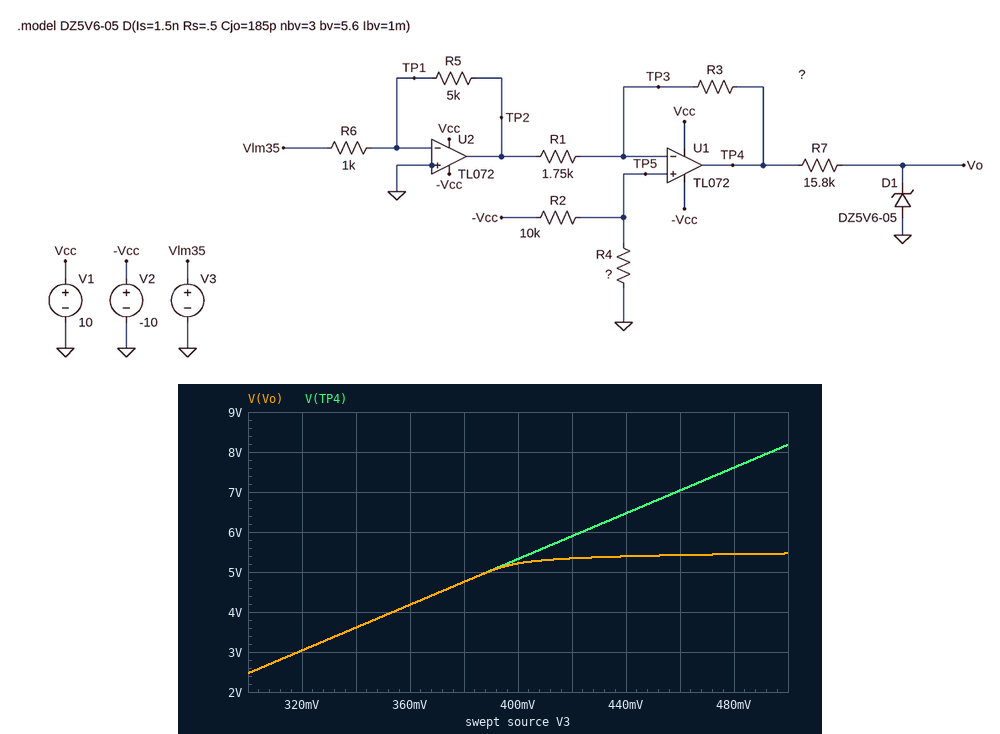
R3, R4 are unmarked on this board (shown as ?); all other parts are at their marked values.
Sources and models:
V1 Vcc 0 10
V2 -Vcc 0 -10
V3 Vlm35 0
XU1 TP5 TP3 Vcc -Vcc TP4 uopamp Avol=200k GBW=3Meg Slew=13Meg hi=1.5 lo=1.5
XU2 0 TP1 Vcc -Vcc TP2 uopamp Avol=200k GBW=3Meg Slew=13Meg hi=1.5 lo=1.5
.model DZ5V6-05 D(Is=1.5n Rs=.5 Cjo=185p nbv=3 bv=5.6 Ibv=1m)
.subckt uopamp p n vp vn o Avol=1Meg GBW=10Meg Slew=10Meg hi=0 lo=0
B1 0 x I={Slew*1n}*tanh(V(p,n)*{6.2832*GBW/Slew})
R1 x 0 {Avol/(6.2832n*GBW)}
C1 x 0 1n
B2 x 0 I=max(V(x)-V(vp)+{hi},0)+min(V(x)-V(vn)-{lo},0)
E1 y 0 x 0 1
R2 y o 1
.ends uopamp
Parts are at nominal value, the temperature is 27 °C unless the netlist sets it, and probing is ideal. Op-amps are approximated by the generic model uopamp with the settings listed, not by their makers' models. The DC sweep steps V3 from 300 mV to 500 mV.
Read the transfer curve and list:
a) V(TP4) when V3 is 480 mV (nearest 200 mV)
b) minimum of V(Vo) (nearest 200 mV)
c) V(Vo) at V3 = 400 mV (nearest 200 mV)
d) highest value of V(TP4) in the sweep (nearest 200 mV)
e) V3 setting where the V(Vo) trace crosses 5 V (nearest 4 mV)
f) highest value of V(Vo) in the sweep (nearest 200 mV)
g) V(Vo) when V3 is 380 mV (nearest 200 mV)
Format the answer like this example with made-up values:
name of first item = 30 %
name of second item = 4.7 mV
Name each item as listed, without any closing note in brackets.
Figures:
V(TP4) when V3 is 480 mV = 7.6 V
minimum of V(Vo) = 2.4 V
V(Vo) at V3 = 400 mV = 5.2 V
highest value of V(TP4) in the sweep = 8.2 V
V3 setting where the V(Vo) trace crosses 5 V = 388 mV
highest value of V(Vo) in the sweep = 5.4 V
V(Vo) when V3 is 380 mV = 4.8 V
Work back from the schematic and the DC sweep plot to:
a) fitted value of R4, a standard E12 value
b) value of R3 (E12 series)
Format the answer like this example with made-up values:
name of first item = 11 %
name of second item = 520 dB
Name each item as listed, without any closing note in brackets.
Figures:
fitted value of R4, a standard E12 value = 1 kΩ
value of R3 = 10 kΩ
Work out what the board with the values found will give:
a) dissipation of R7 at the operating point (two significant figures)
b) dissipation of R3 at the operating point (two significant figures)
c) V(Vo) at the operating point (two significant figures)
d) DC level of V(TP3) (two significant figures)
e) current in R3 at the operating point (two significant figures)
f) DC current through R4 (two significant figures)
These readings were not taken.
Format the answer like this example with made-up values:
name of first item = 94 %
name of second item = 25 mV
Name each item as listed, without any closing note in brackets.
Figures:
dissipation of R7 at the operating point = 2.1 mW
dissipation of R3 at the operating point = 2.7 mW
V(Vo) at the operating point = -320 mV
DC level of V(TP3) = -910 mV
current in R3 at the operating point = 520 µA
DC current through R4 = 910 µA
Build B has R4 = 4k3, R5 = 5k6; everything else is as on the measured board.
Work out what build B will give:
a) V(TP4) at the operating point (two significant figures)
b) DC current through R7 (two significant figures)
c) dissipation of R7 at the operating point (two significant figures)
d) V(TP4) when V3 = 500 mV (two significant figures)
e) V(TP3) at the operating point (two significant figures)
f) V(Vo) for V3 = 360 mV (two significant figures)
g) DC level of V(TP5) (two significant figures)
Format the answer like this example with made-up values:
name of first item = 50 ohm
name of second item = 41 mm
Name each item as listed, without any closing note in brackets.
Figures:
V(TP4) at the operating point = -8.5 V
DC current through R7 = 520 µA
dissipation of R7 at the operating point = 4.2 mW
V(TP4) when V3 = 500 mV = -4.2 V
V(TP3) at the operating point = -1.3 V
V(Vo) for V3 = 360 mV = -330 mV
DC level of V(TP5) = -3.0 V
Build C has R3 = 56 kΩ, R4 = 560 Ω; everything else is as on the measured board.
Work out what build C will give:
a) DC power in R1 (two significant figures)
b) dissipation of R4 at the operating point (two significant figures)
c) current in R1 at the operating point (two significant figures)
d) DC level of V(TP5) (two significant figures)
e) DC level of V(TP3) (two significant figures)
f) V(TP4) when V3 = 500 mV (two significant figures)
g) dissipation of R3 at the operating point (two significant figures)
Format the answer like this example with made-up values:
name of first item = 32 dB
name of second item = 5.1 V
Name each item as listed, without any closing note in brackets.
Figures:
DC power in R1 = 38 µW
dissipation of R4 at the operating point = 500 µW
current in R1 at the operating point = 150 µA
DC level of V(TP5) = -530 mV
DC level of V(TP3) = -260 mV
V(TP4) when V3 = 500 mV = 8.5 V
dissipation of R3 at the operating point = 1.2 mW
